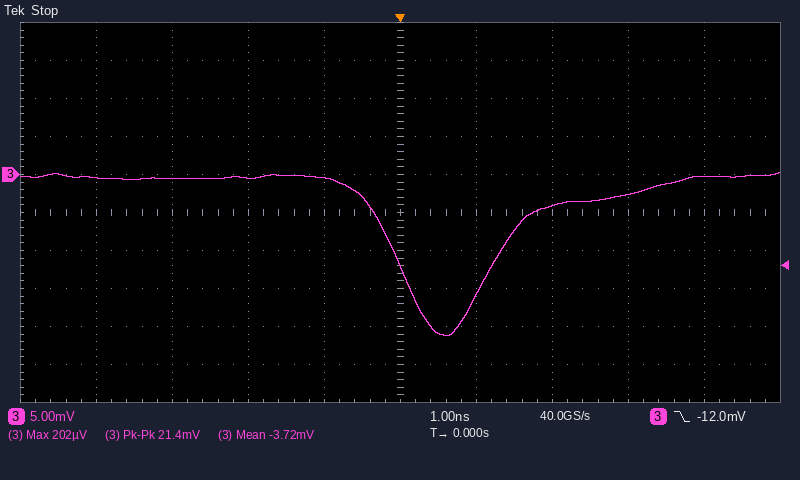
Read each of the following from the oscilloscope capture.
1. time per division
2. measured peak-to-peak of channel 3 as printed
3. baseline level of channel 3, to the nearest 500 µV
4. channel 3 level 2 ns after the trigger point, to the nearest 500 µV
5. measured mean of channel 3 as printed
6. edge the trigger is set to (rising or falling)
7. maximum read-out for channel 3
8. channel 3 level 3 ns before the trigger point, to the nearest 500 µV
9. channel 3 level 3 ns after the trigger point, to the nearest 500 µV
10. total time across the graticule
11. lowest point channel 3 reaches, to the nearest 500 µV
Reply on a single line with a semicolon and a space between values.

1 ns; 21.4 mV; -500 µV; -4.0 mV; -3.72 mV; falling; 202 µV; -500 µV; -2.5 mV; 10 ns; -21.0 mV
